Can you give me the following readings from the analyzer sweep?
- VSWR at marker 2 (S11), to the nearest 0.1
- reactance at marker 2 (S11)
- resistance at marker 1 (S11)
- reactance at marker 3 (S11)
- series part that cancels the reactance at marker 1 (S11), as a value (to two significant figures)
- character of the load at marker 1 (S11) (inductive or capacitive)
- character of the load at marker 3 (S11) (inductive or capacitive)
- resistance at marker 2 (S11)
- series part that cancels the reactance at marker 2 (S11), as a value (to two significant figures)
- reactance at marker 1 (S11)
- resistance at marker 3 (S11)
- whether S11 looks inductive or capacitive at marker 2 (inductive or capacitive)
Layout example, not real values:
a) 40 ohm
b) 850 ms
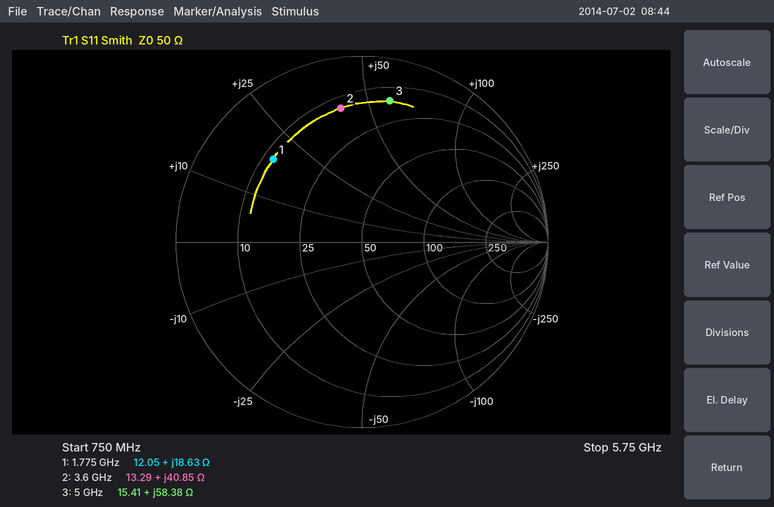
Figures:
a) 6.4
b) +40.85 Ω
c) 12.05 Ω
d) +58.38 Ω
e) 4.8 pF
f) inductive
g) inductive
h) 13.29 Ω
i) 1.1 pF
j) +18.63 Ω
k) 15.41 Ω
l) inductive
